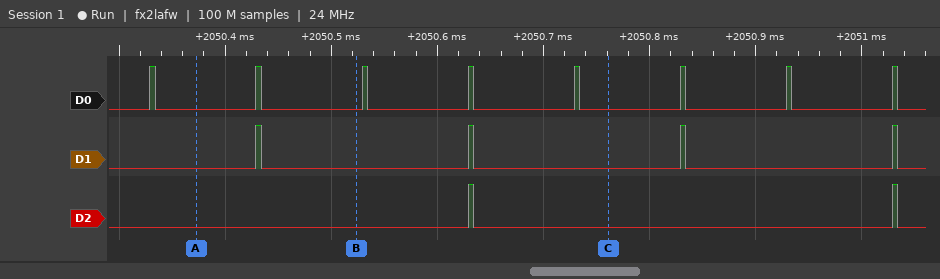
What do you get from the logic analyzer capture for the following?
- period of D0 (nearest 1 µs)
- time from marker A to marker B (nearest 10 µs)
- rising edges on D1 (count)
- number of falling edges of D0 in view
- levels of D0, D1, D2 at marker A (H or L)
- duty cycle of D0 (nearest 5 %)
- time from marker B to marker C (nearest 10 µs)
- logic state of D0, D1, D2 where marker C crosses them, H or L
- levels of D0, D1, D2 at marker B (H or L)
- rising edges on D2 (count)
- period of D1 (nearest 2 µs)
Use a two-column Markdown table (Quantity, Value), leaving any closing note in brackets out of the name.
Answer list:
| Quantity | Value |
|---|---|
| period of D0 | 100 µs |
| time from marker A to marker B | 150 µs |
| rising edges on D1 | 4 |
| number of falling edges of D0 in view | 8 |
| levels of D0, D1, D2 at marker A | D0=L, D1=L, D2=L |
| duty cycle of D0 | 5 % |
| time from marker B to marker C | 240 µs |
| logic state of D0, D1, D2 where marker C crosses them, H or L | D0=L, D1=L, D2=L |
| levels of D0, D1, D2 at marker B | D0=L, D1=L, D2=L |
| rising edges on D2 | 2 |
| period of D1 | 200 µs |
